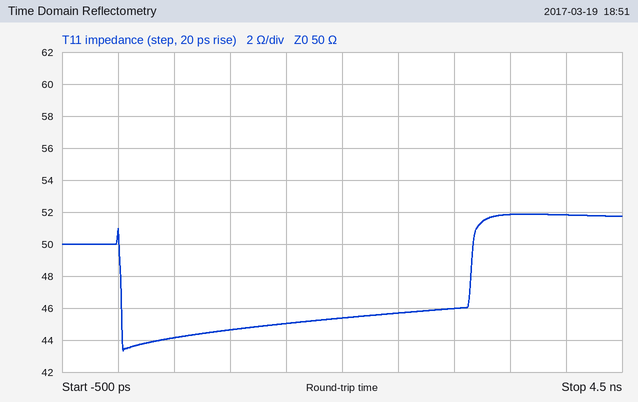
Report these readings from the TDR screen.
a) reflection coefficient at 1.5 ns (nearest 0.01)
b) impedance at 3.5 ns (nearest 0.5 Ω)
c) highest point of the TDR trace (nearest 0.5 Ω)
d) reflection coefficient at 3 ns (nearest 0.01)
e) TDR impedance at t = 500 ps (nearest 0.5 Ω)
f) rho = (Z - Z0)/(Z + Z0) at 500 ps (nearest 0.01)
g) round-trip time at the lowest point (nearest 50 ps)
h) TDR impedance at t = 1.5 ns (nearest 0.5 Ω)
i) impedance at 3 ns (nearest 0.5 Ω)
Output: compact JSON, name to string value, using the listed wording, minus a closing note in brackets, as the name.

{"reflection coefficient at 1.5 ns": "-0.05", "impedance at 3.5 ns": "52.0 Ω", "highest point of the TDR trace": "52.0 Ω", "reflection coefficient at 3 ns": "-0.04", "TDR impedance at t = 500 ps": "44.0 Ω", "rho = (Z - Z0)/(Z + Z0) at 500 ps": "-0.06", "round-trip time at the lowest point": "50 ps", "TDR impedance at t = 1.5 ns": "45.0 Ω", "impedance at 3 ns": "46.0 Ω"}
